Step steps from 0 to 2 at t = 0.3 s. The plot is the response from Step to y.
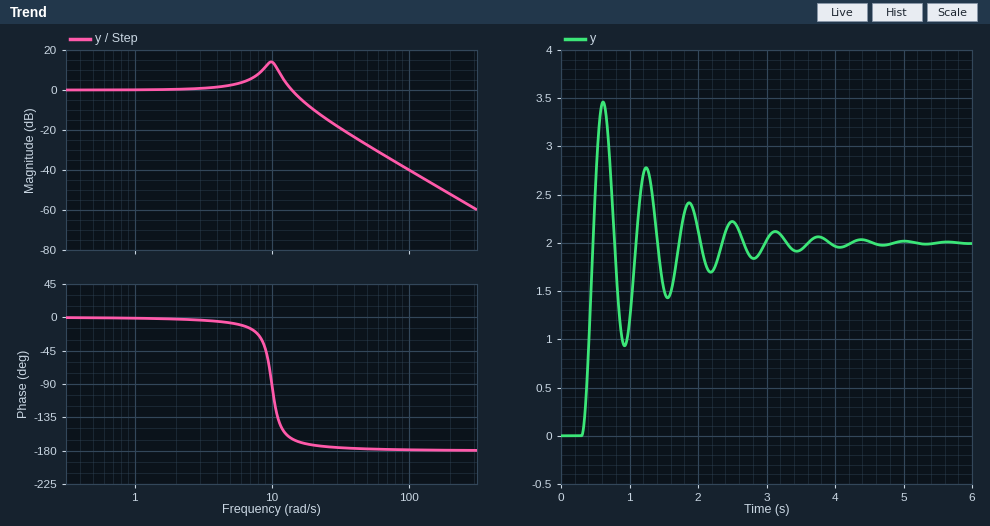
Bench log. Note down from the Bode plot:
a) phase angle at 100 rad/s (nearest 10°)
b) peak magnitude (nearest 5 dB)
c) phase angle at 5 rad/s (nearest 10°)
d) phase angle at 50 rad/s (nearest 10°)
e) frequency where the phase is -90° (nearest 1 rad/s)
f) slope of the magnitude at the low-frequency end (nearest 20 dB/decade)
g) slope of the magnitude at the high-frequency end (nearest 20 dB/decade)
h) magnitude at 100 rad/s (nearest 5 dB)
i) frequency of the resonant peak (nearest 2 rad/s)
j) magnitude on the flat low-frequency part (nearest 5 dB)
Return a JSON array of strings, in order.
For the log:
["-180°", "15 dB", "-10°", "-180°", "10 rad/s", "0 dB/decade", "-40 dB/decade", "-40 dB", "10 rad/s", "0 dB"]
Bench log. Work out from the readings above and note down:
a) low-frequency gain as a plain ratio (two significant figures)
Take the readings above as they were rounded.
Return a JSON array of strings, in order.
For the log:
["1.0"]
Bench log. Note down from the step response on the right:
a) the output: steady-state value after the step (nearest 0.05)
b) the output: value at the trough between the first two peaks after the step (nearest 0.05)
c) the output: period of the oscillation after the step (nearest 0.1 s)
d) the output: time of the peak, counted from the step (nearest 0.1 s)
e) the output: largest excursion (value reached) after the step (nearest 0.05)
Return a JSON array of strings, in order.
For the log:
["2.00", "0.95", "0.6 s", "0.3 s", "3.45"]
